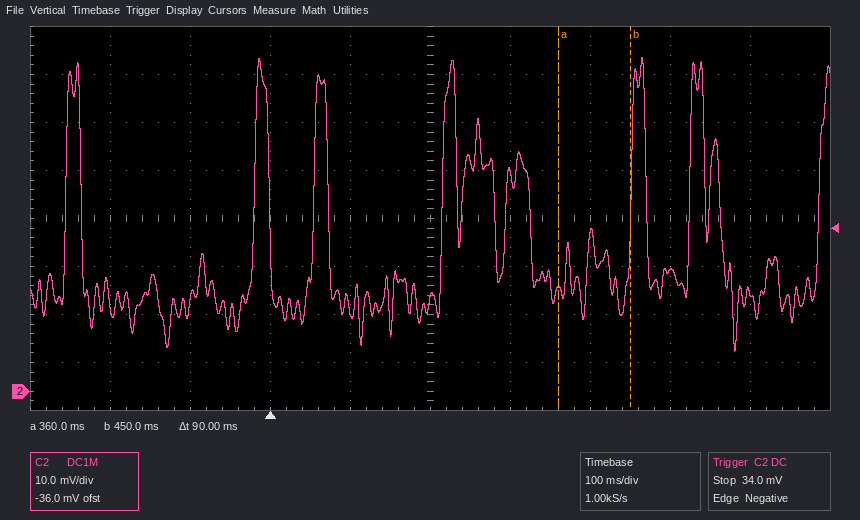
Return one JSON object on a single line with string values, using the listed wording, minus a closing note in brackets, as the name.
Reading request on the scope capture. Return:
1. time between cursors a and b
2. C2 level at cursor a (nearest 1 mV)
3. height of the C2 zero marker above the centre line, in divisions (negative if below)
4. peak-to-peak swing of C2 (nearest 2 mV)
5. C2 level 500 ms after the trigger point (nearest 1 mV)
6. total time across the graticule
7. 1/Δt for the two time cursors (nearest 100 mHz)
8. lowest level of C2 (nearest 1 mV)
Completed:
{"time between cursors a and b": "90 ms", "C2 level at cursor a": "21 mV", "height of the C2 zero marker above the centre line, in divisions": "-3.6 div", "peak-to-peak swing of C2": "62 mV", "C2 level 500 ms after the trigger point": "25 mV", "total time across the graticule": "1 s", "1/Δt for the two time cursors": "11.1 Hz", "lowest level of C2": "8 mV"}
